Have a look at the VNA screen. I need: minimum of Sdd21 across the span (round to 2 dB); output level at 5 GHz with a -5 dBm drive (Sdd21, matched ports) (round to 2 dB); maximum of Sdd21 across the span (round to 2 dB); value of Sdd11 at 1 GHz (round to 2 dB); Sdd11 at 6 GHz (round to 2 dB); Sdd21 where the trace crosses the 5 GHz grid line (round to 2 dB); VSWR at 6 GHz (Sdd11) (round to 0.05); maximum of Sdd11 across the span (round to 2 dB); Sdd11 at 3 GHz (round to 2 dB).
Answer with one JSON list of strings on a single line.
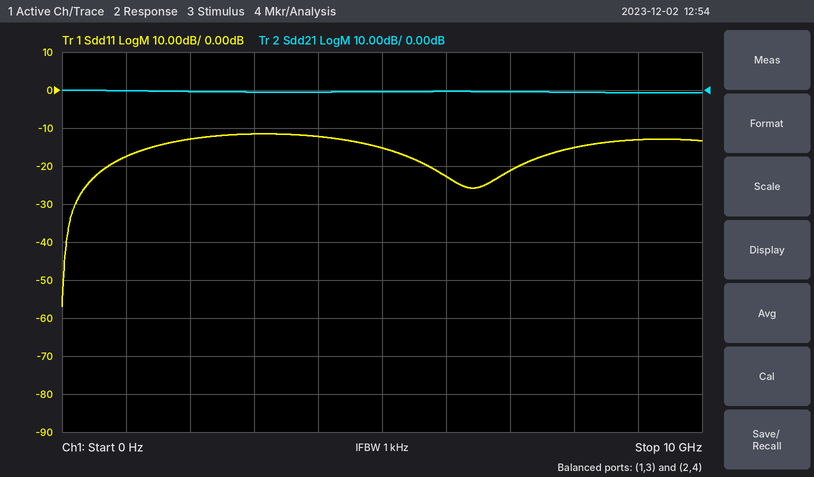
["0 dB", "-6 dBm", "0 dB", "-18 dB", "-22 dB", "0 dB", "1.15", "-12 dB", "-12 dB"]
